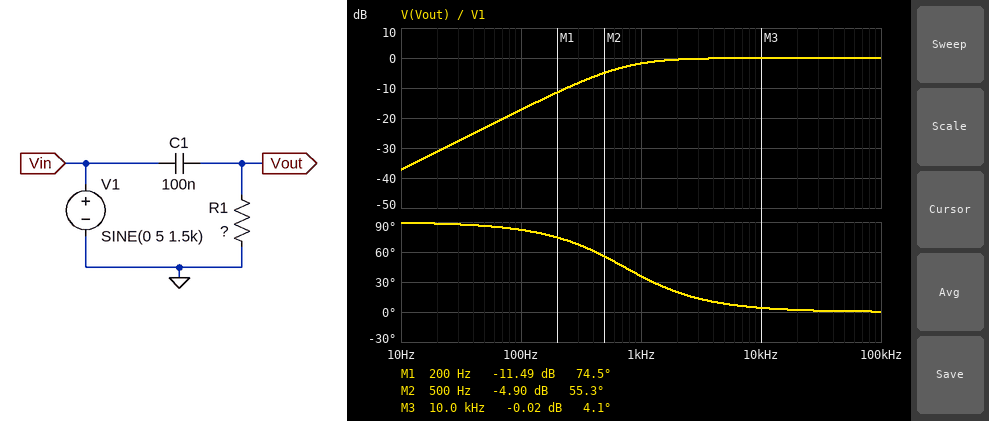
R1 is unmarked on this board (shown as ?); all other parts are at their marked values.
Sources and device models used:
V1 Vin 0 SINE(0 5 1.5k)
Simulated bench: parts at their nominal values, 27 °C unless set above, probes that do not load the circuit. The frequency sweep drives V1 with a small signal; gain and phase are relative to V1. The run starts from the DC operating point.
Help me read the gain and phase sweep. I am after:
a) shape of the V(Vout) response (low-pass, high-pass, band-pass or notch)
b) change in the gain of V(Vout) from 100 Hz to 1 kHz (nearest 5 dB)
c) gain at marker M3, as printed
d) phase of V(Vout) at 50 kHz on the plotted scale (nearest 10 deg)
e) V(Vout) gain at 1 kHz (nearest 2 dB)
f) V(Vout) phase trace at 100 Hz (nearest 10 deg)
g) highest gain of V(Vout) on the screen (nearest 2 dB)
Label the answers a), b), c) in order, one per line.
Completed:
a) high-pass
b) 15 dB
c) -0.02 dB
d) 0 deg
e) -2 dB
f) 80 deg
g) 0 dB
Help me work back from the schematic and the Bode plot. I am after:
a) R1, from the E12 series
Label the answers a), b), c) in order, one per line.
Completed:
a) 2.2 kΩ
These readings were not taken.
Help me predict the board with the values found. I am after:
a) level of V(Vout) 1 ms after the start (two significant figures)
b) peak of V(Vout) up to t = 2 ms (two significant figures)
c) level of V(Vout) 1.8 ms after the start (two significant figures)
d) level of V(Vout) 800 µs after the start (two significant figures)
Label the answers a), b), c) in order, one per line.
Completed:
a) -2.0 V
b) 4.5 V
c) -4.5 V
d) 4.4 V
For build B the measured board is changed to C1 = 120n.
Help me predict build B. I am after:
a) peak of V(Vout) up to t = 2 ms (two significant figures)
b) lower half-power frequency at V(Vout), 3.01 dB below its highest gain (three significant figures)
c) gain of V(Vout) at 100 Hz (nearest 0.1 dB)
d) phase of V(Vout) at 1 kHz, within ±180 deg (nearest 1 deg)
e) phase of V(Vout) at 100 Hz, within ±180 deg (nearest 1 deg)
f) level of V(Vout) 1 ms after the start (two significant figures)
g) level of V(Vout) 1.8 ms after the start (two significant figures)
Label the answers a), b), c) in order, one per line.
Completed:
a) 4.6 V
b) 603 Hz
c) -15.7 dB
d) 31 deg
e) 81 deg
f) -1.8 V
g) -4.6 V
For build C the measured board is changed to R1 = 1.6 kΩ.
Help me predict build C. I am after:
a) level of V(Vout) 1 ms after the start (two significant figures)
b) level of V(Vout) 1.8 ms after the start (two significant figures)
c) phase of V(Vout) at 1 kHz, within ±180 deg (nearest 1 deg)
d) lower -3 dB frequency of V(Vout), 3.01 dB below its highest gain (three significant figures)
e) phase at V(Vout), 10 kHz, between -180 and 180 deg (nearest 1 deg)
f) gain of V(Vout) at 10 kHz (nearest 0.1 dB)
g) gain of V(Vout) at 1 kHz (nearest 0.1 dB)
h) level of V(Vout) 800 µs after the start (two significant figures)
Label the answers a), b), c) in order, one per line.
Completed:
a) -2.3 V
b) -4.0 V
c) 45 deg
d) 995 Hz
e) 6 deg
f) 0 dB
g) -3.0 dB
h) 4.0 V
